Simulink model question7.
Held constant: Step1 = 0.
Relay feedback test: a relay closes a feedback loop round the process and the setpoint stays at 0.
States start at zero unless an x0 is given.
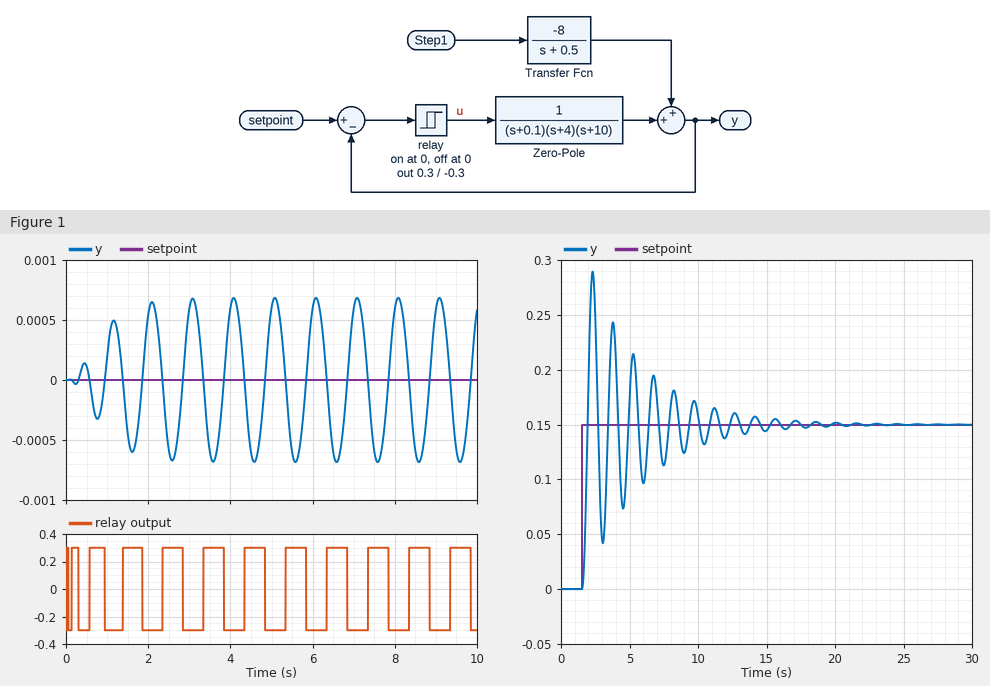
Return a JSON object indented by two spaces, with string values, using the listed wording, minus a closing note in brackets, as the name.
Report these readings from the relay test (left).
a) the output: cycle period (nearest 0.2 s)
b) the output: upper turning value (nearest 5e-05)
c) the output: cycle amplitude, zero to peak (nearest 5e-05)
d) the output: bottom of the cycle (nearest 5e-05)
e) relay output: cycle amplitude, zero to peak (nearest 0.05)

{
  "the output: cycle period": "1.0 s",
  "the output: upper turning value": "0.00070",
  "the output: cycle amplitude, zero to peak": "0.00070",
  "the output: bottom of the cycle": "-0.00070",
  "relay output: cycle amplitude, zero to peak": "0.30"
}
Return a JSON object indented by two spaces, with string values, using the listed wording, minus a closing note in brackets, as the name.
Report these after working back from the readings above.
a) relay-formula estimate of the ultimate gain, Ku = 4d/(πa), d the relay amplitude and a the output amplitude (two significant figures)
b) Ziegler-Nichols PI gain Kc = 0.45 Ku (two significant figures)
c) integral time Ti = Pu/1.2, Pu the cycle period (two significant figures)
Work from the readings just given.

{
  "relay-formula estimate of the ultimate gain, Ku = 4d/(πa), d the relay amplitude and a the output amplitude": "550",
  "Ziegler-Nichols PI gain Kc = 0.45 Ku": "250",
  "integral time Ti = Pu/1.2, Pu the cycle period": "0.83 s"
}
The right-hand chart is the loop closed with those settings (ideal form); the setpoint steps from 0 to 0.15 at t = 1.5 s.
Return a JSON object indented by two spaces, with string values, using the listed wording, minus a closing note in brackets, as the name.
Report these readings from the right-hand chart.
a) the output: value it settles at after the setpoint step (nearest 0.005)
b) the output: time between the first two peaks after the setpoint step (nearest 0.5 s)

{
  "the output: value it settles at after the setpoint step": "0.150",
  "the output: time between the first two peaks after the setpoint step": "1.5 s"
}
